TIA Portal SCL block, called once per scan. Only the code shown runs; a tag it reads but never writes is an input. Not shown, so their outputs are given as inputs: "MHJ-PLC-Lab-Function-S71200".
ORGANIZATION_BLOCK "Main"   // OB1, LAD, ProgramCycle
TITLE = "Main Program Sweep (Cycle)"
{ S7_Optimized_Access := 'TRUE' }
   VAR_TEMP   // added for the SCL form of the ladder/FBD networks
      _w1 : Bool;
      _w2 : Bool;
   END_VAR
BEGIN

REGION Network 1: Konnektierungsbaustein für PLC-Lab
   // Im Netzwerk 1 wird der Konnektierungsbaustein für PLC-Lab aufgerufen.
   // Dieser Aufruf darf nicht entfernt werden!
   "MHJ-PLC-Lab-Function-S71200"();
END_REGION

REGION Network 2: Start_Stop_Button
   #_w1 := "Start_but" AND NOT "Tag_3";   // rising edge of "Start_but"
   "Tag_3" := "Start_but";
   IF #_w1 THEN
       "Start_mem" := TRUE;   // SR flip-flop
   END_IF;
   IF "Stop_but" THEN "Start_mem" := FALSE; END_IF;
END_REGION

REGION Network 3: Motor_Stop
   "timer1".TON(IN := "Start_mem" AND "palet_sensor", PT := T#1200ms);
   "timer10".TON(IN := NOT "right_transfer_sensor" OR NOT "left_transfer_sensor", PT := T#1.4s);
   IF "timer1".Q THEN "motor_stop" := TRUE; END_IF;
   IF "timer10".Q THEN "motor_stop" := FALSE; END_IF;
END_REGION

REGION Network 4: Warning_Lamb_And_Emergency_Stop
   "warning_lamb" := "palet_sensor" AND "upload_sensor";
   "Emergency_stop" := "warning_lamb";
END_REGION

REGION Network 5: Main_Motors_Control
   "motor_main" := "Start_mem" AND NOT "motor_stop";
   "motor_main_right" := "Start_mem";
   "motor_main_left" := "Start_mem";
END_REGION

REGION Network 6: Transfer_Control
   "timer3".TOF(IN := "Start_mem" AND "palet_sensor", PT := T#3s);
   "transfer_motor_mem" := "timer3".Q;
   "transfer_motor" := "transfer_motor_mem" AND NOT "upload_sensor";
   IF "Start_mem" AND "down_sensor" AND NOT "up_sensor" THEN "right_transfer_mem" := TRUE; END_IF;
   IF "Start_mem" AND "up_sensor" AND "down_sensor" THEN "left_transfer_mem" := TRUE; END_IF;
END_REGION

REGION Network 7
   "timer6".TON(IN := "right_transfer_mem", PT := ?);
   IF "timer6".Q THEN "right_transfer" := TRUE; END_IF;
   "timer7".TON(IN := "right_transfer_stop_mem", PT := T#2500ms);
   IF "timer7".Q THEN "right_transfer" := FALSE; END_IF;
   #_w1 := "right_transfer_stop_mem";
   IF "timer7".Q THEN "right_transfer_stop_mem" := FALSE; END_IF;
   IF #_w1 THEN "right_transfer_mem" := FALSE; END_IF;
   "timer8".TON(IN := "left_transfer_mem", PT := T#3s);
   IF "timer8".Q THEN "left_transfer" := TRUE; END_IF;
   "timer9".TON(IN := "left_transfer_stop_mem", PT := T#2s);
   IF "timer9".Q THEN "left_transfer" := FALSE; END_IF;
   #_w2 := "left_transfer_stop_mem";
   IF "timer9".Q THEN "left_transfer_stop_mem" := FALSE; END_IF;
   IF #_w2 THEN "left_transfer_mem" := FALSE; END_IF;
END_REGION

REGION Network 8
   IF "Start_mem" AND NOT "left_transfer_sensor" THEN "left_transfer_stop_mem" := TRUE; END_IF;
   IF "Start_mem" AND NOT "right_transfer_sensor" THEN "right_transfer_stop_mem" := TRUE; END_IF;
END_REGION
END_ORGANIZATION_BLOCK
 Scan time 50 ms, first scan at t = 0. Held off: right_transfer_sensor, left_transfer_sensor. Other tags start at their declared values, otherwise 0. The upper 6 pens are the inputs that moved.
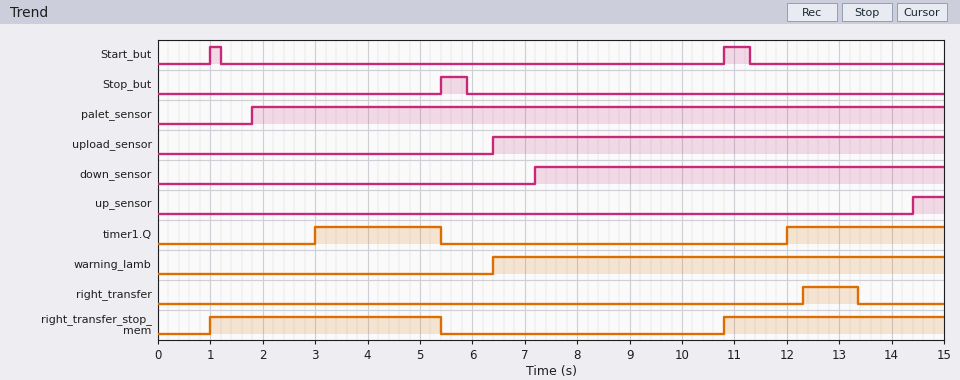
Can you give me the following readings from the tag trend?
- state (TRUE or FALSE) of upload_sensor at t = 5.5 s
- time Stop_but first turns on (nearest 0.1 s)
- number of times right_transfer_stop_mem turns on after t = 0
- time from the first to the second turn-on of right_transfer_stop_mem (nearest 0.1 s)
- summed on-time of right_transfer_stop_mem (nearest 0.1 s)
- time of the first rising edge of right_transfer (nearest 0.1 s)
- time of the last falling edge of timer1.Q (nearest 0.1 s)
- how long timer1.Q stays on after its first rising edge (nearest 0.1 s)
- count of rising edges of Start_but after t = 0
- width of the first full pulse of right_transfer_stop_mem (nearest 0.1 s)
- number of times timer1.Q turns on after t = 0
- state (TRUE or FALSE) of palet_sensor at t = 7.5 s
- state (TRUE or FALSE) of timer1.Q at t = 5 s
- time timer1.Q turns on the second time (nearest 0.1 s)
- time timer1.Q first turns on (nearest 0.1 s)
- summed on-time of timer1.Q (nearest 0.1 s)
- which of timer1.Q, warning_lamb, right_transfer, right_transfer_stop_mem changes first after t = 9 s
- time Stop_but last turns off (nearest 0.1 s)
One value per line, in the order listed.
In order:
FALSE
5.4 s
2
9.8 s
8.6 s
12.3 s
5.4 s
2.4 s
2
4.4 s
2
TRUE
TRUE
12.0 s
3.0 s
5.4 s
right_transfer_stop_mem
5.9 s
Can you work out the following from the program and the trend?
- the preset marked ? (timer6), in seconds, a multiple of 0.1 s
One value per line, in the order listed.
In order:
1.5 s
